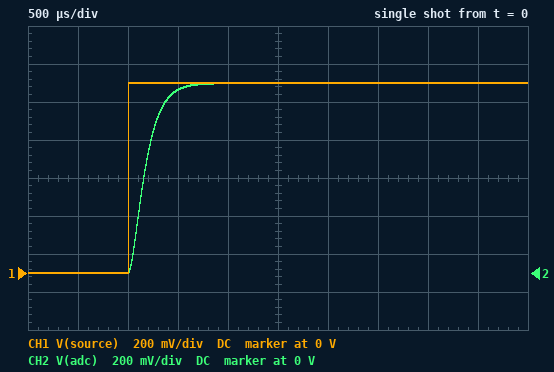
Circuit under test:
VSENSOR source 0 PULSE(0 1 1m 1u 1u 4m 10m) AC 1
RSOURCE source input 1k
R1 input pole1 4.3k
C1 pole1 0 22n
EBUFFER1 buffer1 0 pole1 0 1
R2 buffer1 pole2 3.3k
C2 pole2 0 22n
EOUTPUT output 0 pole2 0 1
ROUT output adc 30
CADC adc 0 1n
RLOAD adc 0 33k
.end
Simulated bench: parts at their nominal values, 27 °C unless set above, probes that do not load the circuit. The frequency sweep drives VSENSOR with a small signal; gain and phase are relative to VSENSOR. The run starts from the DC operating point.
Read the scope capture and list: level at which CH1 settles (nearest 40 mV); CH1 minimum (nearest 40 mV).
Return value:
1.00 V
0 V
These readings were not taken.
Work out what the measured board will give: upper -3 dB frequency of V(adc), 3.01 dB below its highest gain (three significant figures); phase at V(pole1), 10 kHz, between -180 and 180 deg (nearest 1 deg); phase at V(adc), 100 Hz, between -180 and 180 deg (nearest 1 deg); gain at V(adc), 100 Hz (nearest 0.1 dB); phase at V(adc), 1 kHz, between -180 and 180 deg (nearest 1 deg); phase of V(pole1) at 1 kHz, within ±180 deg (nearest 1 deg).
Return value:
1.07 kHz
-82 deg
-7 deg
0 dB
-61 deg
-36 deg
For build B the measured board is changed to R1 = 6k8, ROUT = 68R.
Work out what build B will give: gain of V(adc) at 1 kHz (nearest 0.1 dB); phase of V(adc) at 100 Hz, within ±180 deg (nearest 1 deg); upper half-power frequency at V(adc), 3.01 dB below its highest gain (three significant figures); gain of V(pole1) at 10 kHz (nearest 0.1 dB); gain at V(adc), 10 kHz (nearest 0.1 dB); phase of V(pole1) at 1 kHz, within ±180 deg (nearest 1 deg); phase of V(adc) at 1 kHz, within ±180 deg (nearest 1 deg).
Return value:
-4.2 dB
-9 deg
809 Hz
-20.7 dB
-34.1 dB
-47 deg
-72 deg
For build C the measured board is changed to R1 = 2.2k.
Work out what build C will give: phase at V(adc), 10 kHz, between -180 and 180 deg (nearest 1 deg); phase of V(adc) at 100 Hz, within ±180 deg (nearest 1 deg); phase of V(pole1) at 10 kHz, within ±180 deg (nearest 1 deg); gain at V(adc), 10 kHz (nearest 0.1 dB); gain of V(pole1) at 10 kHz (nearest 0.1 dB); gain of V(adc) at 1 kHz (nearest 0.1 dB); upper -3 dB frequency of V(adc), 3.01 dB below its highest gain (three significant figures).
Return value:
-155 deg
-5 deg
-77 deg
-26.5 dB
-13.1 dB
-1.6 dB
1.43 kHz
